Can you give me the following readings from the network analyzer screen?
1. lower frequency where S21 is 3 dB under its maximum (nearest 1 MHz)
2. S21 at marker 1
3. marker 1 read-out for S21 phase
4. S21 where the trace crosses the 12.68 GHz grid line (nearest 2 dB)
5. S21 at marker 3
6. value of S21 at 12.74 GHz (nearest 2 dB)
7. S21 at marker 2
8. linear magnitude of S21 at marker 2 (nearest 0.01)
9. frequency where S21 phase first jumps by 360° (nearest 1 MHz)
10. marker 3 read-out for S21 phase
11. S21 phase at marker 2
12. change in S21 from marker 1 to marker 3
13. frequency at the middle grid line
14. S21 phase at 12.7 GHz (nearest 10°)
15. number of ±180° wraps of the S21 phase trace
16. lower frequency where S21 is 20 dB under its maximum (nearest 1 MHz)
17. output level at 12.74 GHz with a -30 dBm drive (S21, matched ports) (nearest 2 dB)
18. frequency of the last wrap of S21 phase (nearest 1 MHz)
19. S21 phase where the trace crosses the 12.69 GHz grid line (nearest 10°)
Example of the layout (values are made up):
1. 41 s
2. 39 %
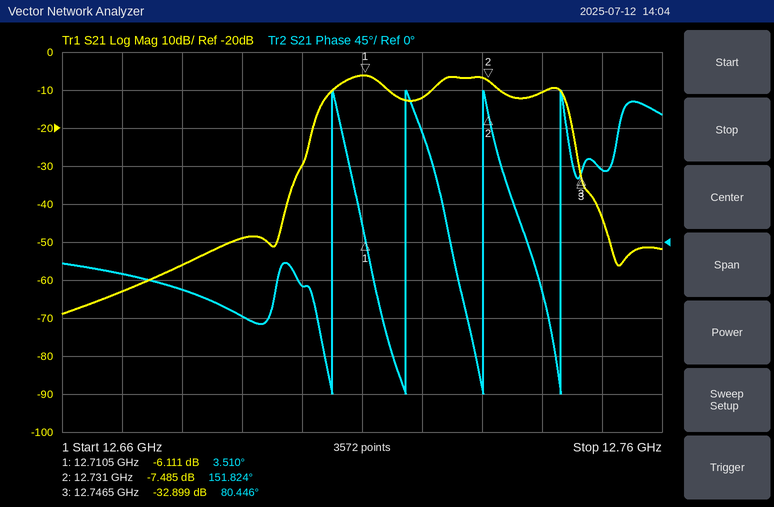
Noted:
1. 12.706 GHz
2. -6.111 dB
3. 3.510°
4. -56 dB
5. -32.899 dB
6. -10 dB
7. -7.485 dB
8. 0.42
9. 12.705 GHz
10. 80.446°
11. 151.824°
12. -26.788 dB
13. 12.71 GHz
14. -50°
15. 4
16. 12.701 GHz
17. -40 dBm
18. 12.743 GHz
19. -90°
